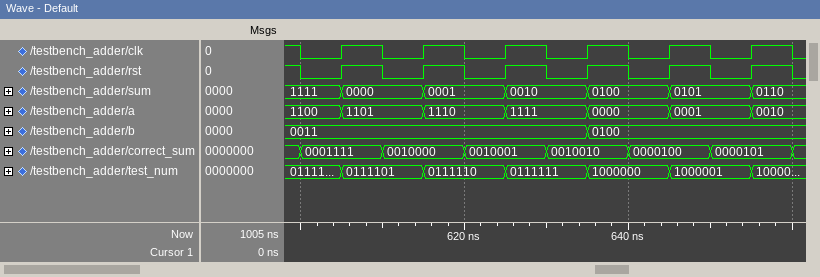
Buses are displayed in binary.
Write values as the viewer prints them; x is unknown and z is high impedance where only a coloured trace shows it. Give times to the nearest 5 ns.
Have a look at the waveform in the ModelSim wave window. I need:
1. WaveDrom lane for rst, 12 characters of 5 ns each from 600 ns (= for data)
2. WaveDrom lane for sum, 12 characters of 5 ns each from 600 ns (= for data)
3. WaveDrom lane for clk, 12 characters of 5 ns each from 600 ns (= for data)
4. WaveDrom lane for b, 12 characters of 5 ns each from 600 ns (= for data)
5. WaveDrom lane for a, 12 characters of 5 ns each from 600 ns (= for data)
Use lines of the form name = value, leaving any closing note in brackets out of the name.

WaveDrom lane for rst, 12 characters of 5 ns each from 600 ns = {name: 'rst', wave: '010101010101'}
WaveDrom lane for sum, 12 characters of 5 ns each from 600 ns = {name: 'sum', wave: '==.=.=.=.=.=', data: '1111 0000 0001 0010 0100 0101 0110'}
WaveDrom lane for clk, 12 characters of 5 ns each from 600 ns = {name: 'clk', wave: '010101010101'}
WaveDrom lane for b, 12 characters of 5 ns each from 600 ns = {name: 'b', wave: '=......=....', data: '0011 0100'}
WaveDrom lane for a, 12 characters of 5 ns each from 600 ns = {name: 'a', wave: '==.=.=.=.=.=', data: '1100 1101 1110 1111 0000 0001 0010'}
